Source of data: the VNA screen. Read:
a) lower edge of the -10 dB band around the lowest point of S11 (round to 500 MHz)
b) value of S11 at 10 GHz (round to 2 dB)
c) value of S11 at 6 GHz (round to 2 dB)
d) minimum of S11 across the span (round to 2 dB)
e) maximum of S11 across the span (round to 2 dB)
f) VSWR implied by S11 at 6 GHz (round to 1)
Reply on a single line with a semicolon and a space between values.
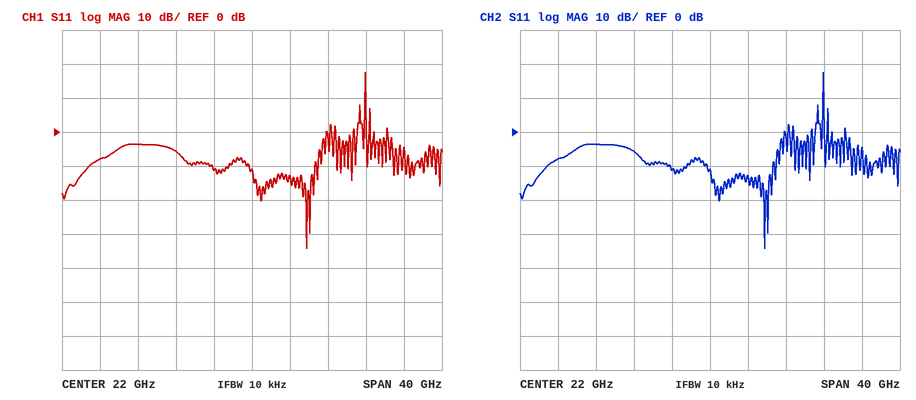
21.5 GHz; -4 dB; -8 dB; -34 dB; 18 dB; 2
